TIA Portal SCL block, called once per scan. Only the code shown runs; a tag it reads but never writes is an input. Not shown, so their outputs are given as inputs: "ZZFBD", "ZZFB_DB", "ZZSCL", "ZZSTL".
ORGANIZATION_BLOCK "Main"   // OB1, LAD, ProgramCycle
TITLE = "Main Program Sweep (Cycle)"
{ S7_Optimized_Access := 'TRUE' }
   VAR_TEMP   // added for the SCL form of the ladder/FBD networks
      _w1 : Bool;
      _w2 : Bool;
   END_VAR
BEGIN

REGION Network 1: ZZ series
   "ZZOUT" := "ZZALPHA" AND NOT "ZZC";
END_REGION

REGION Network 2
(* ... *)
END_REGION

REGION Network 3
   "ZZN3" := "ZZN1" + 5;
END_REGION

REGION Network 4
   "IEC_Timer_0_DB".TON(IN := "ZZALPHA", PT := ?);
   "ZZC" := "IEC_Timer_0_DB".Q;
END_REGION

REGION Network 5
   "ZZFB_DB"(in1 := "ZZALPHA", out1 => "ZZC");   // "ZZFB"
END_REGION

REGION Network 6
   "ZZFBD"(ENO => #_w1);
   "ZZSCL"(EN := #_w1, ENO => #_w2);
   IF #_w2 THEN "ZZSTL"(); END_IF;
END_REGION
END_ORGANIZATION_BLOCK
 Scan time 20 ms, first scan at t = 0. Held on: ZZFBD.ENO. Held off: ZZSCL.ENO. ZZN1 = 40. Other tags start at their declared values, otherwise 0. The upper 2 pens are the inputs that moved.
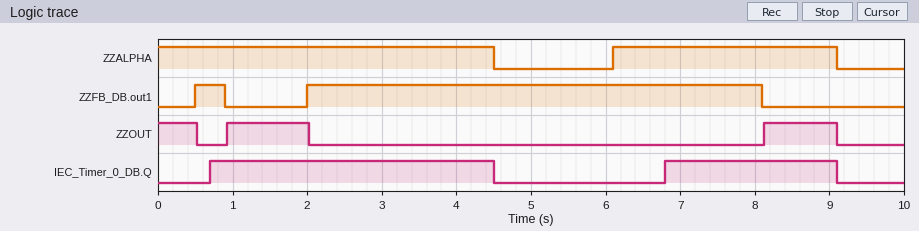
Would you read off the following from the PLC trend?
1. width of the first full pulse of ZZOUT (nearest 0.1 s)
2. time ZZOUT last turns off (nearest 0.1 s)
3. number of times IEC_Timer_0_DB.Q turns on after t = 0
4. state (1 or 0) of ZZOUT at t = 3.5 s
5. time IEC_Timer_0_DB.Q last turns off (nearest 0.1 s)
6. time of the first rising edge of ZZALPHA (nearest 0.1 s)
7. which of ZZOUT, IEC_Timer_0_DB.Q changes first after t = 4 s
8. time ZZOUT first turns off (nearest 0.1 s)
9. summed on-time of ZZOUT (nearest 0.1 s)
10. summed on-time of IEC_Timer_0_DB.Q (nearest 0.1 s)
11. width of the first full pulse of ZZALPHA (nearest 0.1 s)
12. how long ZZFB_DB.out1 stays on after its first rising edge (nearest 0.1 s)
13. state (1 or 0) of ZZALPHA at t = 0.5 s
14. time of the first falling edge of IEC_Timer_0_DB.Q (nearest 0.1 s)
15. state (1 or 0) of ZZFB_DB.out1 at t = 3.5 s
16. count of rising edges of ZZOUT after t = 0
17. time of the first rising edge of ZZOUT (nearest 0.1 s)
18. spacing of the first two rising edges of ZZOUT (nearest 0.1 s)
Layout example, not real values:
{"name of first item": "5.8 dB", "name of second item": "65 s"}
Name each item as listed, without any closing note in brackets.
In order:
{"width of the first full pulse of ZZOUT": "1.1 s", "time ZZOUT last turns off": "9.1 s", "number of times IEC_Timer_0_DB.Q turns on after t = 0": "2", "state (1 or 0) of ZZOUT at t = 3.5 s": "0", "time IEC_Timer_0_DB.Q last turns off": "9.1 s", "time of the first rising edge of ZZALPHA": "6.1 s", "which of ZZOUT, IEC_Timer_0_DB.Q changes first after t = 4 s": "IEC_Timer_0_DB.Q", "time ZZOUT first turns off": "0.5 s", "summed on-time of ZZOUT": "2.6 s", "summed on-time of IEC_Timer_0_DB.Q": "6.1 s", "width of the first full pulse of ZZALPHA": "3.0 s", "how long ZZFB_DB.out1 stays on after its first rising edge": "0.4 s", "state (1 or 0) of ZZALPHA at t = 0.5 s": "1", "time of the first falling edge of IEC_Timer_0_DB.Q": "4.5 s", "state (1 or 0) of ZZFB_DB.out1 at t = 3.5 s": "1", "count of rising edges of ZZOUT after t = 0": "2", "time of the first rising edge of ZZOUT": "0.9 s", "spacing of the first two rising edges of ZZOUT": "7.2 s"}
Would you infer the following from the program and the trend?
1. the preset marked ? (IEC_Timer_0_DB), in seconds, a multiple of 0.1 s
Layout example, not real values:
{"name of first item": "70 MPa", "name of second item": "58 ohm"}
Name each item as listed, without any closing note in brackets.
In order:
{"the preset marked ? (IEC_Timer_0_DB), in seconds, a multiple of 0.1 s": "0.7 s"}
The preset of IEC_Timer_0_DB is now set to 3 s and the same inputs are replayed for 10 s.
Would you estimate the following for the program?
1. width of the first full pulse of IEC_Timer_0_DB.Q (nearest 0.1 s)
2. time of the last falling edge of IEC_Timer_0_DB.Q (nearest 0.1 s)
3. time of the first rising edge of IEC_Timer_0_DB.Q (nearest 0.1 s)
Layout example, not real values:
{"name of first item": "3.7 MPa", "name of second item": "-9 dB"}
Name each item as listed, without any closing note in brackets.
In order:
{"width of the first full pulse of IEC_Timer_0_DB.Q": "1.5 s", "time of the last falling edge of IEC_Timer_0_DB.Q": "4.5 s", "time of the first rising edge of IEC_Timer_0_DB.Q": "3.0 s"}
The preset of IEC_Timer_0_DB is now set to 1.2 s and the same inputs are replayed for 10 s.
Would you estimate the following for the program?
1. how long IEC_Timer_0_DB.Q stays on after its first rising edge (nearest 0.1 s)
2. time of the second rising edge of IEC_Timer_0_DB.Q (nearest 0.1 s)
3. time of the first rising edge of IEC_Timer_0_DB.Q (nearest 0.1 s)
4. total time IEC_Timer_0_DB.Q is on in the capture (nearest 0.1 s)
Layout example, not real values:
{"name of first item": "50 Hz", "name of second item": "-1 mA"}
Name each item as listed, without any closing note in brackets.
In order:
{"how long IEC_Timer_0_DB.Q stays on after its first rising edge": "3.3 s", "time of the second rising edge of IEC_Timer_0_DB.Q": "7.3 s", "time of the first rising edge of IEC_Timer_0_DB.Q": "1.2 s", "total time IEC_Timer_0_DB.Q is on in the capture": "5.1 s"}
